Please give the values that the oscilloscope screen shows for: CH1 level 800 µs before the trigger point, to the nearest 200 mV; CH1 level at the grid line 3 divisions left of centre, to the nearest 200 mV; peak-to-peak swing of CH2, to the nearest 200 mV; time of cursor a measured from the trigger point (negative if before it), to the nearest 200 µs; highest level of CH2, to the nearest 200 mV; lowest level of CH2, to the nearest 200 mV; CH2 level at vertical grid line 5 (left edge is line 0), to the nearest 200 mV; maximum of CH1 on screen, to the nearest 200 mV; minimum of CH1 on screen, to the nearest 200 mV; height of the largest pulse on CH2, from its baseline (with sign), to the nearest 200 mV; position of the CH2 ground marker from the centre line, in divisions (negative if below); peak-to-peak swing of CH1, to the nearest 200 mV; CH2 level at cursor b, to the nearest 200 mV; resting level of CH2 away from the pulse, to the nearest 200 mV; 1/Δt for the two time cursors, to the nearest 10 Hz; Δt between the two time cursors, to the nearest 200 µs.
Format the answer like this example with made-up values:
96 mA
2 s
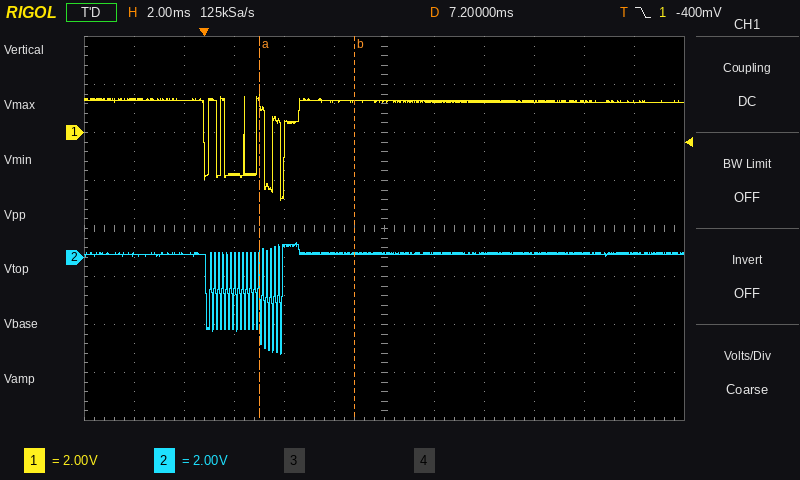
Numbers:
1.4 V
-1.8 V
4.6 V
+2.2 ms
600 mV
-4.0 V
200 mV
1.6 V
-2.8 V
-4.2 V
-0.6 div
4.4 V
200 mV
200 mV
260 Hz
3.8 ms
